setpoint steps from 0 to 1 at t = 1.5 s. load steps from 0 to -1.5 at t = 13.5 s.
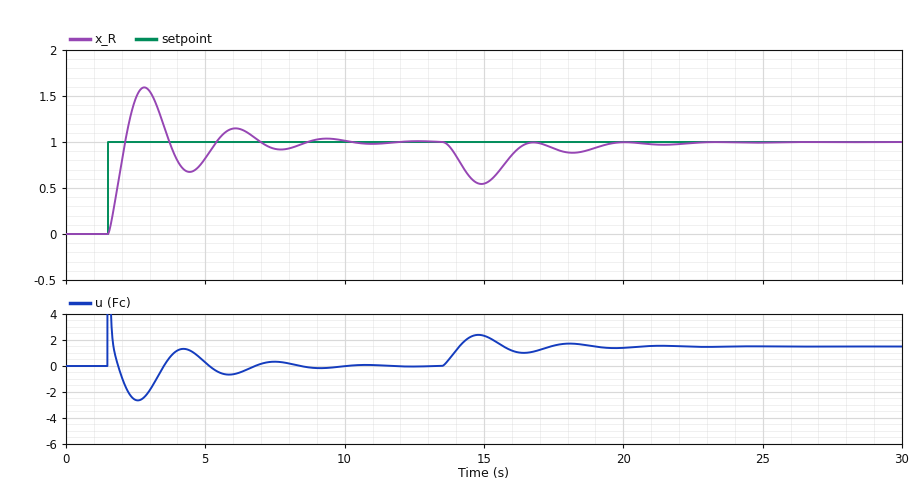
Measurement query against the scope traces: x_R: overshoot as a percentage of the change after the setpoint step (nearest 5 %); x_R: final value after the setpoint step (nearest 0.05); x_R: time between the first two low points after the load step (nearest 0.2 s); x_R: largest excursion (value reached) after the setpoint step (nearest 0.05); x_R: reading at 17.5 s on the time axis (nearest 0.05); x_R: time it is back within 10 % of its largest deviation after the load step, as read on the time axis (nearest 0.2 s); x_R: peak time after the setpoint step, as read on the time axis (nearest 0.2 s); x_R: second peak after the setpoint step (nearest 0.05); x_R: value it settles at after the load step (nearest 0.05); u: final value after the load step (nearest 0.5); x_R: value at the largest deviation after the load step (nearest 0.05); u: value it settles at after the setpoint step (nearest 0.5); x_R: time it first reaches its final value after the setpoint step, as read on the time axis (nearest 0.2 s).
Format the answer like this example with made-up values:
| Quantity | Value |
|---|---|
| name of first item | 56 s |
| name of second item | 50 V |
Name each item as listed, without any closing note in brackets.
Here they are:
| Quantity | Value |
|---|---|
| x_R: overshoot as a percentage of the change after the setpoint step | 60 % |
| x_R: final value after the setpoint step | 1.00 |
| x_R: time between the first two low points after the load step | 3.2 s |
| x_R: largest excursion (value reached) after the setpoint step | 1.60 |
| x_R: reading at 17.5 s on the time axis | 0.95 |
| x_R: time it is back within 10 % of its largest deviation after the load step, as read on the time axis | 19.2 s |
| x_R: peak time after the setpoint step, as read on the time axis | 2.8 s |
| x_R: second peak after the setpoint step | 1.15 |
| x_R: value it settles at after the load step | 1.00 |
| u: final value after the load step | 1.5 |
| x_R: value at the largest deviation after the load step | 0.55 |
| u: value it settles at after the setpoint step | 0.0 |
| x_R: time it first reaches its final value after the setpoint step, as read on the time axis | 2.2 s |
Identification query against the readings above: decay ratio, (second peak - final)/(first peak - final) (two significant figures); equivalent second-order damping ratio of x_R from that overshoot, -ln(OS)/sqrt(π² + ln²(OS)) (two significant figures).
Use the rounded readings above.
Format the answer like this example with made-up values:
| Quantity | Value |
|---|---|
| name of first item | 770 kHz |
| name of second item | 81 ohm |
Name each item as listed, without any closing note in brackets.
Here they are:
| Quantity | Value |
|---|---|
| decay ratio, (second peak - final)/(first peak - final) | 0.25 |
| equivalent second-order damping ratio of x_R from that overshoot, -ln(OS)/sqrt(π² + ln²(OS)) | 0.16 |
